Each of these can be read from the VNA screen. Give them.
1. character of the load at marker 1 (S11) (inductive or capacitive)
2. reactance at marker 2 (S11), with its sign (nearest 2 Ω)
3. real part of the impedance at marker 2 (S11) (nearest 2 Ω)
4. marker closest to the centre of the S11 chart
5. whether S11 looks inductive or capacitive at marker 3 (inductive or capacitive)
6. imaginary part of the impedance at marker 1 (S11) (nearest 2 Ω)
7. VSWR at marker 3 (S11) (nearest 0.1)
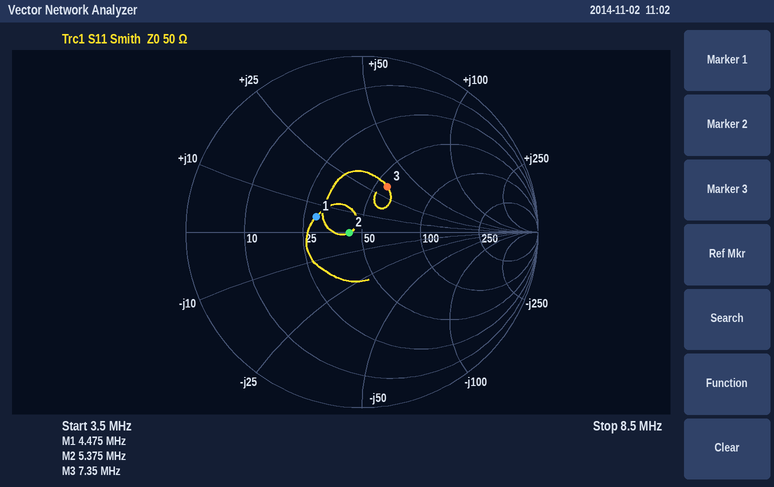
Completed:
inductive
0 Ω
44 Ω
marker 2
inductive
+6 Ω
1.8
